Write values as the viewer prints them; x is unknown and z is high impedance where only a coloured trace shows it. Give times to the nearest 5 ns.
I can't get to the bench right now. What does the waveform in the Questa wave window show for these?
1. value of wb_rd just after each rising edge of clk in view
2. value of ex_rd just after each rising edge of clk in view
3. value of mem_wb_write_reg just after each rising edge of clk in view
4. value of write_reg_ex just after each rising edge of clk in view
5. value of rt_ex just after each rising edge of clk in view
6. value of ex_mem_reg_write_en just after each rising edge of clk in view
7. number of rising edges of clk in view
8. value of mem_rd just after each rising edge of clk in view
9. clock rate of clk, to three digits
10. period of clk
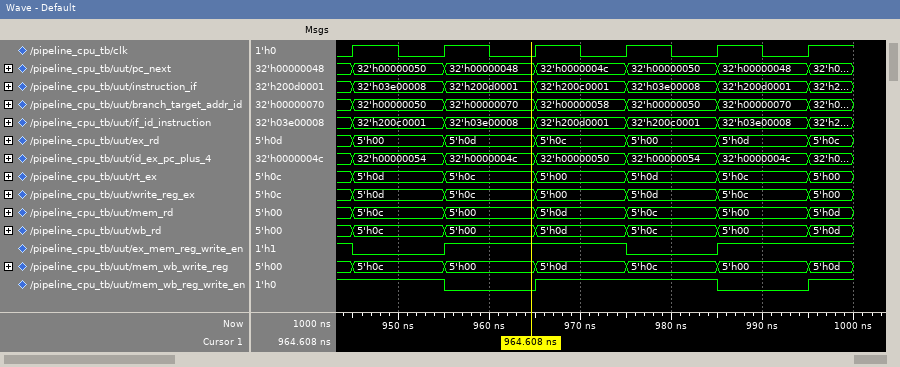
5'h0c, 5'h00, 5'h0d, 5'h0c, 5'h00, 5'h0d
5'h00, 5'h0d, 5'h0c, 5'h00, 5'h0d, 5'h0c
5'h0c, 5'h00, 5'h0d, 5'h0c, 5'h00, 5'h0d
5'h0d, 5'h0c, 5'h00, 5'h0d, 5'h0c, 5'h00
5'h0d, 5'h0c, 5'h00, 5'h0d, 5'h0c, 5'h00
0 1 1 0 1 1
6
5'h0c, 5'h00, 5'h0d, 5'h0c, 5'h00, 5'h0d
100 MHz
10 ns
